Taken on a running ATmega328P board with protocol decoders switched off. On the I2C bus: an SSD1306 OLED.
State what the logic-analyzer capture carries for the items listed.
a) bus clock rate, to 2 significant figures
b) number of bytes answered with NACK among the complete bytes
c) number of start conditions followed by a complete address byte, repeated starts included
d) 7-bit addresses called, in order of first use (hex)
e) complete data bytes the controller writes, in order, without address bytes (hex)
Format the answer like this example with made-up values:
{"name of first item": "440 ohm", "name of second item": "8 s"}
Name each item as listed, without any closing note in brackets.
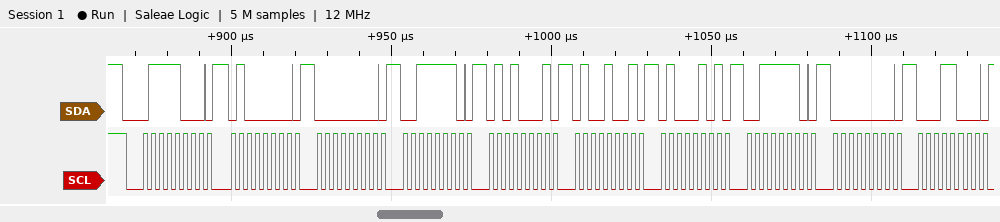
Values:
{"bus clock rate, to 2 significant figures": "400 kHz", "number of bytes answered with NACK among the complete bytes": "0", "number of start conditions followed by a complete address byte, repeated starts included": "1", "7-bit addresses called, in order of first use": "0x3C", "complete data bytes the controller writes, in order, without address bytes": "40 00 3E 51 49 45 3E 00 18"}
